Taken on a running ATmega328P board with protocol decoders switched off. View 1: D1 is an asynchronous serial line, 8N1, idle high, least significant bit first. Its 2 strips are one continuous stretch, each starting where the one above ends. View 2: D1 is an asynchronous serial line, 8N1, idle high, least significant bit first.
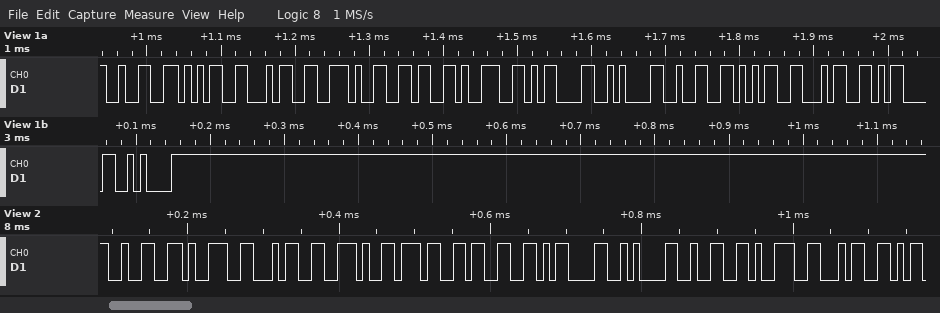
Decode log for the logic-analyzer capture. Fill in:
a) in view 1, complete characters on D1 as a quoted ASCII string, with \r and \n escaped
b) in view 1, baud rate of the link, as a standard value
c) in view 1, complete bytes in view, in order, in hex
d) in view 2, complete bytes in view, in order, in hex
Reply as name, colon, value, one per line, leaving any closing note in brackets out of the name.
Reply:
in view 1, complete characters on D1 as a quoted ASCII string, with \r and \n escaped: "254.69\r\n254\r\n"
in view 1, baud rate of the link, as a standard value: 115200 baud
in view 1, complete bytes in view, in order, in hex: 32 35 34 2E 36 39 0D 0A 32 35 34 0D 0A
in view 2, complete bytes in view, in order, in hex: 32 39 34 2E 37 33 0D 0A 32 39 34
